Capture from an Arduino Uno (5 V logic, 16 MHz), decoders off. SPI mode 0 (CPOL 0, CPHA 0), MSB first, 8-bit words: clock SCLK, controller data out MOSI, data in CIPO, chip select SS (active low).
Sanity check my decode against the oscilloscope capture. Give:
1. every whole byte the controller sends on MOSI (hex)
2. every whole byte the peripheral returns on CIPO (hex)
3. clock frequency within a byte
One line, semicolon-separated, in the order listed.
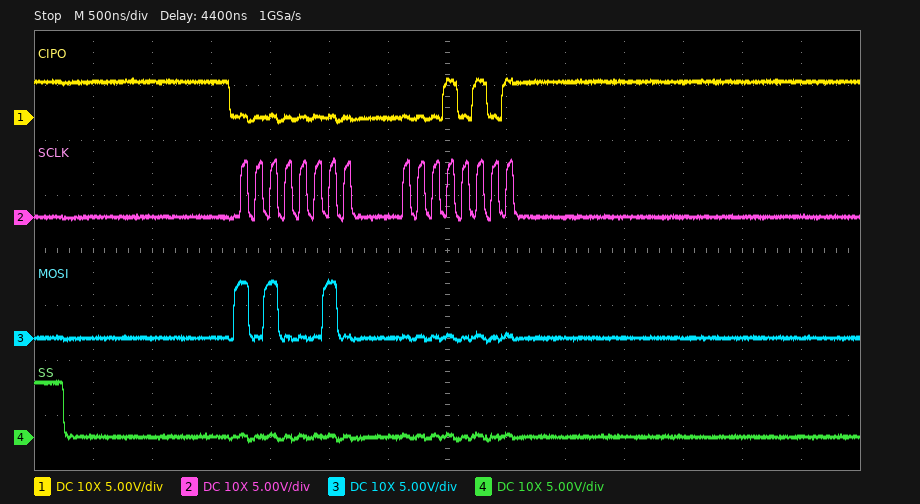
0xA2 0x00; 0x00 0x15; 8 MHz
